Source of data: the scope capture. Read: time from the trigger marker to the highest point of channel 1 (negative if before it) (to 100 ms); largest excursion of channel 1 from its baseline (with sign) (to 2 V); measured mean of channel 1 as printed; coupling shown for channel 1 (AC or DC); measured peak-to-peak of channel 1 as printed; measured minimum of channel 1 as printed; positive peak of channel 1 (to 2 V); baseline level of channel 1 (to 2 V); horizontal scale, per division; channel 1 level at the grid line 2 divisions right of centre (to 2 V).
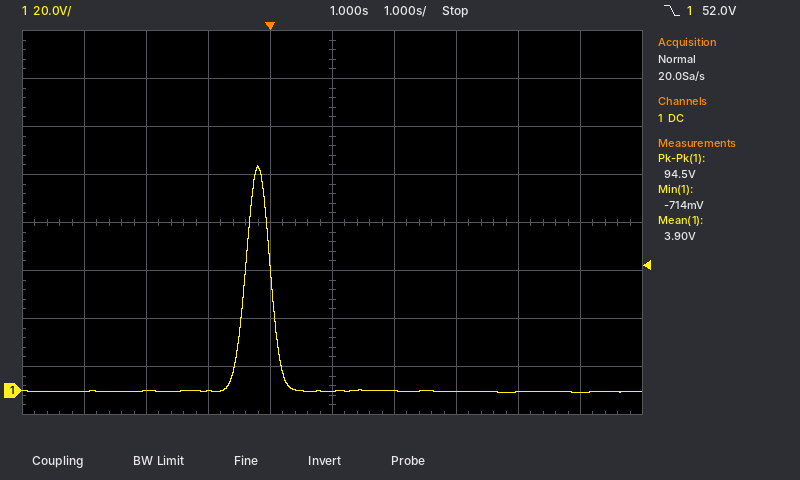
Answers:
-200 ms
+94 V
3.90 V
DC
94.5 V
-714 mV
94 V
0 V
1 s
0 V
